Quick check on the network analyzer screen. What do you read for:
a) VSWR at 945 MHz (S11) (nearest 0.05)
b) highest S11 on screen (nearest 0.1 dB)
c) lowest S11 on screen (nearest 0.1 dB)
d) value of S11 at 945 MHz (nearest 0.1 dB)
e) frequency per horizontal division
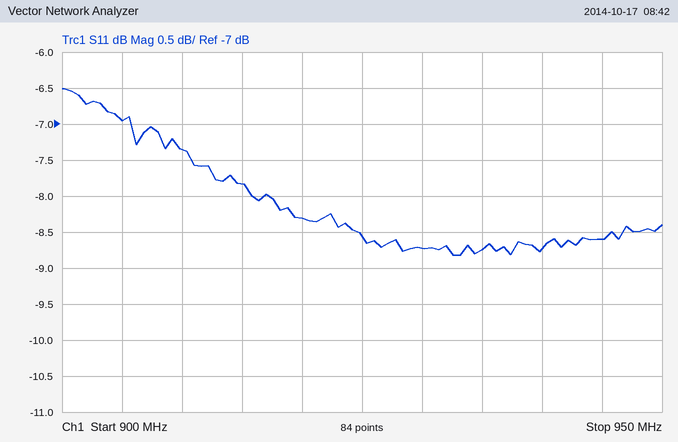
2.20
-6.5 dB
-8.8 dB
-8.6 dB
5 MHz
